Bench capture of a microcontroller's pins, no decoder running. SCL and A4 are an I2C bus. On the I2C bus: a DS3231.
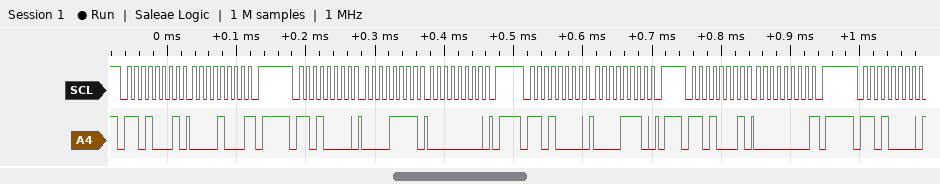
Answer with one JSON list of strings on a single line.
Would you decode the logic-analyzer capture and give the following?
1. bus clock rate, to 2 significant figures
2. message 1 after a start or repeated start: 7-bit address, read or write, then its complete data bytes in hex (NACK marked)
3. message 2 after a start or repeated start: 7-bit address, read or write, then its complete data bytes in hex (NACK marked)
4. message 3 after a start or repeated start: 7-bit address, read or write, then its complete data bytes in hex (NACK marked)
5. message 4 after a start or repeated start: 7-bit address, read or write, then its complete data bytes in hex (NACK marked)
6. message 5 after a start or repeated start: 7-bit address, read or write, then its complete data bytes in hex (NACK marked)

["100 kHz", "0x68 read: 08 NACK", "0x68 write: 0F 00", "0x68 write: 0E", "0x68 read: 00 NACK", "0x68 write"]
